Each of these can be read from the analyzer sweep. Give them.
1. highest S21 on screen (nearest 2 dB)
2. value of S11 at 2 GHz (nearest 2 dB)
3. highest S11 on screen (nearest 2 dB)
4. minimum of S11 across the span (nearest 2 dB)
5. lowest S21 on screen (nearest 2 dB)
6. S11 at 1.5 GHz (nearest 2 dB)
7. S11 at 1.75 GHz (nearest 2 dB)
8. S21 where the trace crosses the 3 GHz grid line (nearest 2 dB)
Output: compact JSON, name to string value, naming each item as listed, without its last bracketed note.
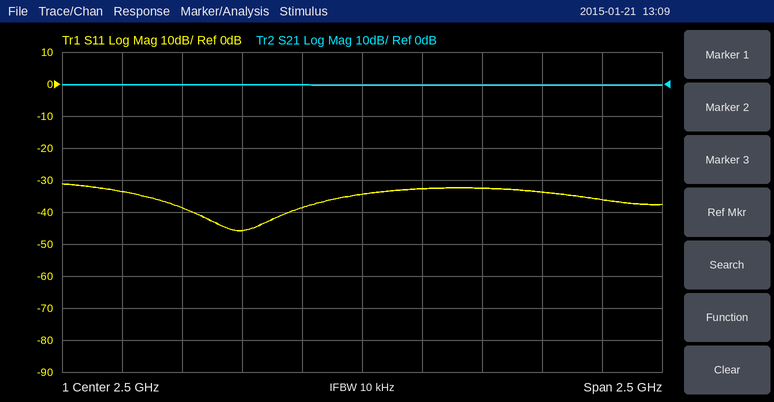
{"highest S21 on screen": "0 dB", "value of S11 at 2 GHz": "-46 dB", "highest S11 on screen": "-32 dB", "minimum of S11 across the span": "-46 dB", "lowest S21 on screen": "0 dB", "S11 at 1.5 GHz": "-34 dB", "S11 at 1.75 GHz": "-38 dB", "S21 where the trace crosses the 3 GHz grid line": "0 dB"}
